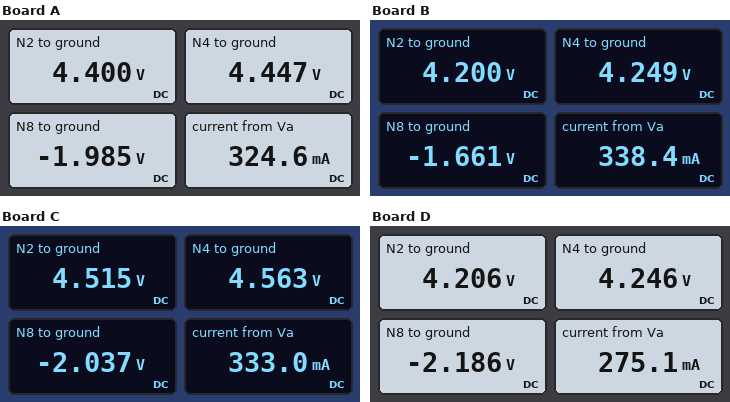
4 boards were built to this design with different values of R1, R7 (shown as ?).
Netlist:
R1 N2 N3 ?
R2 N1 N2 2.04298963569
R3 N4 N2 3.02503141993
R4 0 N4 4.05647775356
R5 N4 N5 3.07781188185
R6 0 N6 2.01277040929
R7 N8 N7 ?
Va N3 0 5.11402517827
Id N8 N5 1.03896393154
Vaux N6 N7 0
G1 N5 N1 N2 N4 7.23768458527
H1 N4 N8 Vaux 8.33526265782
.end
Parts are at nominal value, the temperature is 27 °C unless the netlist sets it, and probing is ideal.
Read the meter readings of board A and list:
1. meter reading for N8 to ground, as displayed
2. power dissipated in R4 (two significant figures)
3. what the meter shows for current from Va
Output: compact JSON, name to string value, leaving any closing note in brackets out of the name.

{"meter reading for N8 to ground, as displayed": "-1.985 V", "power dissipated in R4": "4.9 W", "what the meter shows for current from Va": "324.6 mA"}
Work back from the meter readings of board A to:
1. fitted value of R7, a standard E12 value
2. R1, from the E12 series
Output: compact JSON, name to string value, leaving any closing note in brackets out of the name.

{"fitted value of R7, a standard E12 value": "0.56 Ω", "R1, from the E12 series": "2.2 Ω"}
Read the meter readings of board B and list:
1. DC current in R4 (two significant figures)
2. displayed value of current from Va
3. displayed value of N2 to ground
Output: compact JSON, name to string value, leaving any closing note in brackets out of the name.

{"DC current in R4": "1.0 A", "displayed value of current from Va": "338.4 mA", "displayed value of N2 to ground": "4.200 V"}
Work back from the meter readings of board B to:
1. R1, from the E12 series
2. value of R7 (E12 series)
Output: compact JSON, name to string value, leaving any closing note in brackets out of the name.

{"R1, from the E12 series": "2.7 Ω", "value of R7": "0.33 Ω"}
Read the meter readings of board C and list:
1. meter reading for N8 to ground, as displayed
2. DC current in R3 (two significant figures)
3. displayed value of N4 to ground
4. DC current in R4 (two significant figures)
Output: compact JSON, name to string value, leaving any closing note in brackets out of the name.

{"meter reading for N8 to ground, as displayed": "-2.037 V", "DC current in R3": "16 mA", "displayed value of N4 to ground": "4.563 V", "DC current in R4": "1.1 A"}
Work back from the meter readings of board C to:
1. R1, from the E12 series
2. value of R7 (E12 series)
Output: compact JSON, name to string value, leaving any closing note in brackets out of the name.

{"R1, from the E12 series": "1.8 Ω", "value of R7": "0.56 Ω"}
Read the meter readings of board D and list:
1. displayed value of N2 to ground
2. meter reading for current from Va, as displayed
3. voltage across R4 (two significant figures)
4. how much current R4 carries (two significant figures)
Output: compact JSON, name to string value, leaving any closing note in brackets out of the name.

{"displayed value of N2 to ground": "4.206 V", "meter reading for current from Va, as displayed": "275.1 mA", "voltage across R4": "4.2 V", "how much current R4 carries": "1.0 A"}
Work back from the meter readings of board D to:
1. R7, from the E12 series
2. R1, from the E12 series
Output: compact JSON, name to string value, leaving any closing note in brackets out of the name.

{"R7, from the E12 series": "0.82 Ω", "R1, from the E12 series": "3.3 Ω"}
